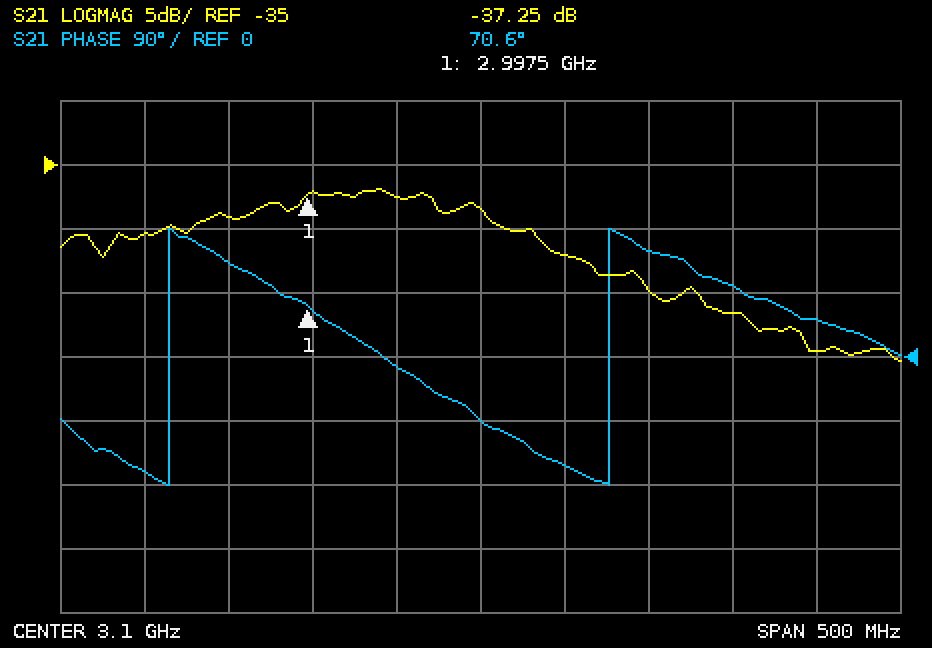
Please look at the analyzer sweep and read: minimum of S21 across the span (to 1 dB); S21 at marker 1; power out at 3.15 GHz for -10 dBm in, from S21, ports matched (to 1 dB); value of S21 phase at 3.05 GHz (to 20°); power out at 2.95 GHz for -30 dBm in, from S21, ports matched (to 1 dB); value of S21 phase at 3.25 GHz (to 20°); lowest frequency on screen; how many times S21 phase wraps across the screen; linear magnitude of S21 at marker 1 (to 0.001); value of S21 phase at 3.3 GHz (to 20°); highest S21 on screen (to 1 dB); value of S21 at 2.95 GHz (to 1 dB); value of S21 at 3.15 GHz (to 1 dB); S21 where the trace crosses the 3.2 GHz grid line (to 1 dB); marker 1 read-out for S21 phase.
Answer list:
-50 dB
-37.25 dB
-52 dBm
-20°
-69 dBm
100°
2.85 GHz
2
0.014
60°
-37 dB
-39 dB
-42 dB
-45 dB
70.6°
